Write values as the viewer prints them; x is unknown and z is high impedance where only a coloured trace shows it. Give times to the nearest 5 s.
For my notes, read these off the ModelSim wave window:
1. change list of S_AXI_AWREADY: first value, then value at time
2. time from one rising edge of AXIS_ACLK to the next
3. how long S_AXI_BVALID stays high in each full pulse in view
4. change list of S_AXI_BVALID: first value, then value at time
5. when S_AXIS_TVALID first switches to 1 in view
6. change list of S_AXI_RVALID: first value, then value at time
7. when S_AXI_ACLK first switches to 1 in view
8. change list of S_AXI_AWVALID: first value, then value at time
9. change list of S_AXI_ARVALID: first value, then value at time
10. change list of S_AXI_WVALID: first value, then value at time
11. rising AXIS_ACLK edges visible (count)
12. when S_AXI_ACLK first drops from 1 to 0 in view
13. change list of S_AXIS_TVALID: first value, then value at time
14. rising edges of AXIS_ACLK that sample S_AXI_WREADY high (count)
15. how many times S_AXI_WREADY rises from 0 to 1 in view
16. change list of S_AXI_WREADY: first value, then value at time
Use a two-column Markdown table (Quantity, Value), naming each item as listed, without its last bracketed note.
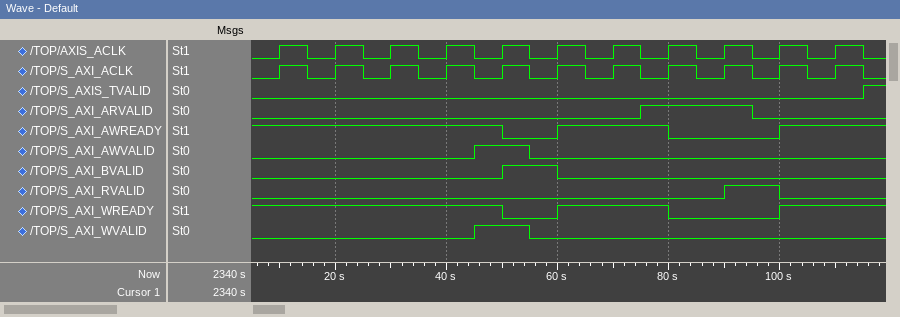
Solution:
| Quantity | Value |
|---|---|
| change list of S_AXI_AWREADY: first value, then value at time | 1, 0 at 50 s, 1 at 60 s, 0 at 80 s, 1 at 100 s |
| time from one rising edge of AXIS_ACLK to the next | 10 s |
| how long S_AXI_BVALID stays high in each full pulse in view | 10 s |
| change list of S_AXI_BVALID: first value, then value at time | 0, 1 at 50 s, 0 at 60 s |
| when S_AXIS_TVALID first switches to 1 in view | 115 s |
| change list of S_AXI_RVALID: first value, then value at time | 0, 1 at 90 s, 0 at 100 s |
| when S_AXI_ACLK first switches to 1 in view | 10 s |
| change list of S_AXI_AWVALID: first value, then value at time | 0, 1 at 45 s, 0 at 55 s |
| change list of S_AXI_ARVALID: first value, then value at time | 0, 1 at 75 s, 0 at 95 s |
| change list of S_AXI_WVALID: first value, then value at time | 0, 1 at 45 s, 0 at 55 s |
| rising AXIS_ACLK edges visible | 11 |
| when S_AXI_ACLK first drops from 1 to 0 in view | 15 s |
| change list of S_AXIS_TVALID: first value, then value at time | 0, 1 at 115 s |
| rising edges of AXIS_ACLK that sample S_AXI_WREADY high | 8 |
| how many times S_AXI_WREADY rises from 0 to 1 in view | 2 |
| change list of S_AXI_WREADY: first value, then value at time | 1, 0 at 50 s, 1 at 60 s, 0 at 80 s, 1 at 100 s |
